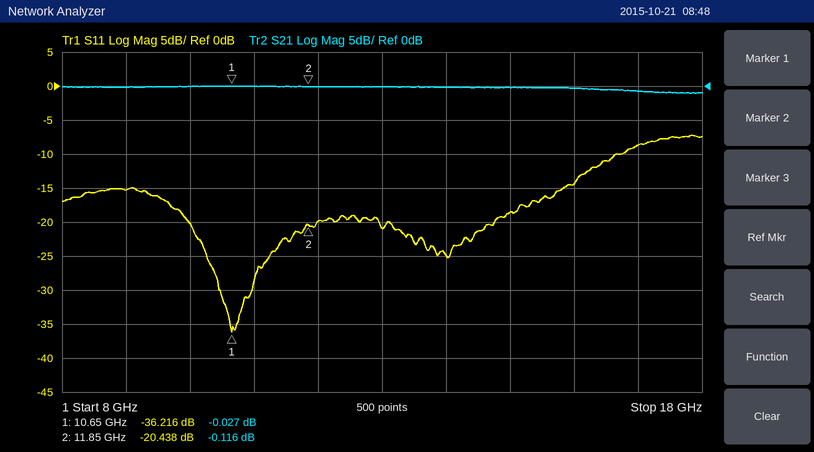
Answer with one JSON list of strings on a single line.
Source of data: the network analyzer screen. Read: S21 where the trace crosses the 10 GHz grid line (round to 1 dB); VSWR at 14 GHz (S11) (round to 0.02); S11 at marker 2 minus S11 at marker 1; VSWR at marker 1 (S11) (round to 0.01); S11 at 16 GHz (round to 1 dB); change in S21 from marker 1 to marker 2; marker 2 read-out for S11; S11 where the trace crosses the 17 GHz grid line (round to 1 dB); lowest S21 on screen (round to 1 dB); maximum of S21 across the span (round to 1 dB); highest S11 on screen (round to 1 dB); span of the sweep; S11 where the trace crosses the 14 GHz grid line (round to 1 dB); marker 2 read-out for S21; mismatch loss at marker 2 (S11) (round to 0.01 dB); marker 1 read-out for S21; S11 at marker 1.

["0 dB", "1.12", "15.778 dB", "1.03", "-14 dB", "-0.089 dB", "-20.438 dB", "-9 dB", "-1 dB", "0 dB", "-7 dB", "10 GHz", "-25 dB", "-0.116 dB", "0.04 dB", "-0.027 dB", "-36.216 dB"]
